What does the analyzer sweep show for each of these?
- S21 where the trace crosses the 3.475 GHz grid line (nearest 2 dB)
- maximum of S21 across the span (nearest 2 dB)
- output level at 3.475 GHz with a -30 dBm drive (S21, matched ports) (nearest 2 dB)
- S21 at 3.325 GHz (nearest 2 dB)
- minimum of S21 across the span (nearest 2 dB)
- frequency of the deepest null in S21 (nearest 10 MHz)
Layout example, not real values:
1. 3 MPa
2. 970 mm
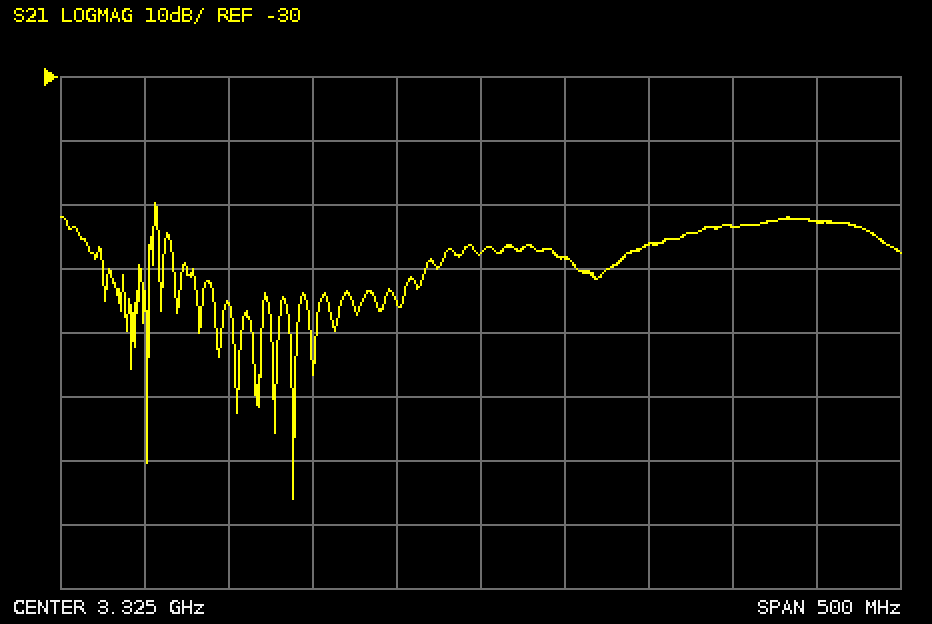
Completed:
1. -54 dB
2. -50 dB
3. -84 dBm
4. -58 dB
5. -96 dB
6. 3.21 GHz
